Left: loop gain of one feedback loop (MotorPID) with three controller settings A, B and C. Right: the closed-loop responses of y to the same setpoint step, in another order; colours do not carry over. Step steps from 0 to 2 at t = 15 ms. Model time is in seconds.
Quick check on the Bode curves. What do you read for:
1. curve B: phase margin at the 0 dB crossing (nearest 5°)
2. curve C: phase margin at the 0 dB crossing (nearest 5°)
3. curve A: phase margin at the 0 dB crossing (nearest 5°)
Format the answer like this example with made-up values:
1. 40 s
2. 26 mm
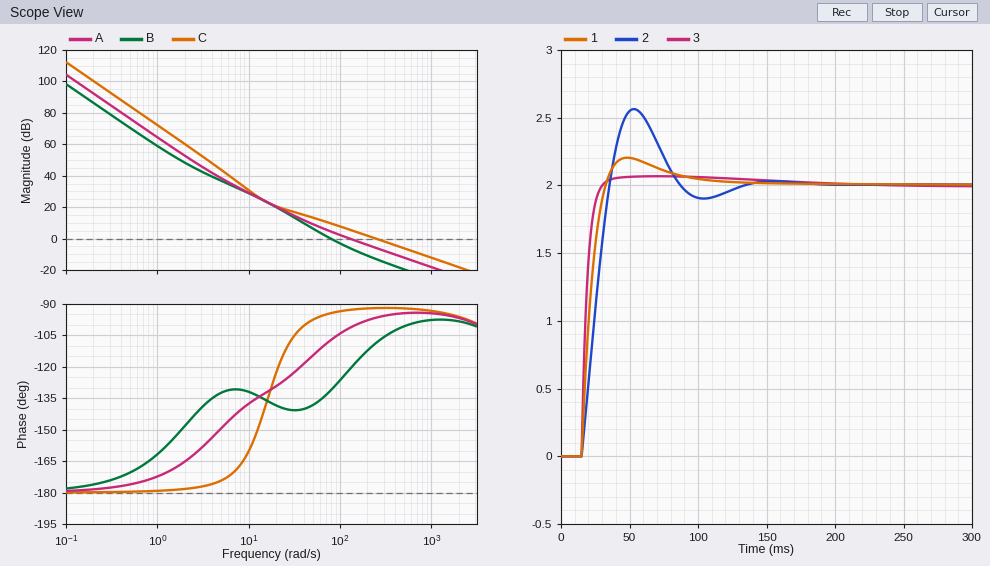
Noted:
1. 50°
2. 90°
3. 80°
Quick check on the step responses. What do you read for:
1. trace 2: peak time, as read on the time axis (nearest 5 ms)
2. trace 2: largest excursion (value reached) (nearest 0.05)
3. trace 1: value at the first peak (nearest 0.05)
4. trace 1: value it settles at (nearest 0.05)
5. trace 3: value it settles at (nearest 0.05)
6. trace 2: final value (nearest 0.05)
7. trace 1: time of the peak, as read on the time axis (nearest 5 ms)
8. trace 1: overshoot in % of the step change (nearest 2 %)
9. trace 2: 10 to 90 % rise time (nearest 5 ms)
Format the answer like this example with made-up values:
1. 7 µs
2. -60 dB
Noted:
1. 55 ms
2. 2.55
3. 2.20
4. 2.00
5. 2.00
6. 2.00
7. 50 ms
8. 10 %
9. 15 ms
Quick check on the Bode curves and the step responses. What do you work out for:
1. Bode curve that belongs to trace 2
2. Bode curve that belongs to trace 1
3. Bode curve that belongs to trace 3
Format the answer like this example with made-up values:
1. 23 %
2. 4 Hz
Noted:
1. B
2. A
3. C
